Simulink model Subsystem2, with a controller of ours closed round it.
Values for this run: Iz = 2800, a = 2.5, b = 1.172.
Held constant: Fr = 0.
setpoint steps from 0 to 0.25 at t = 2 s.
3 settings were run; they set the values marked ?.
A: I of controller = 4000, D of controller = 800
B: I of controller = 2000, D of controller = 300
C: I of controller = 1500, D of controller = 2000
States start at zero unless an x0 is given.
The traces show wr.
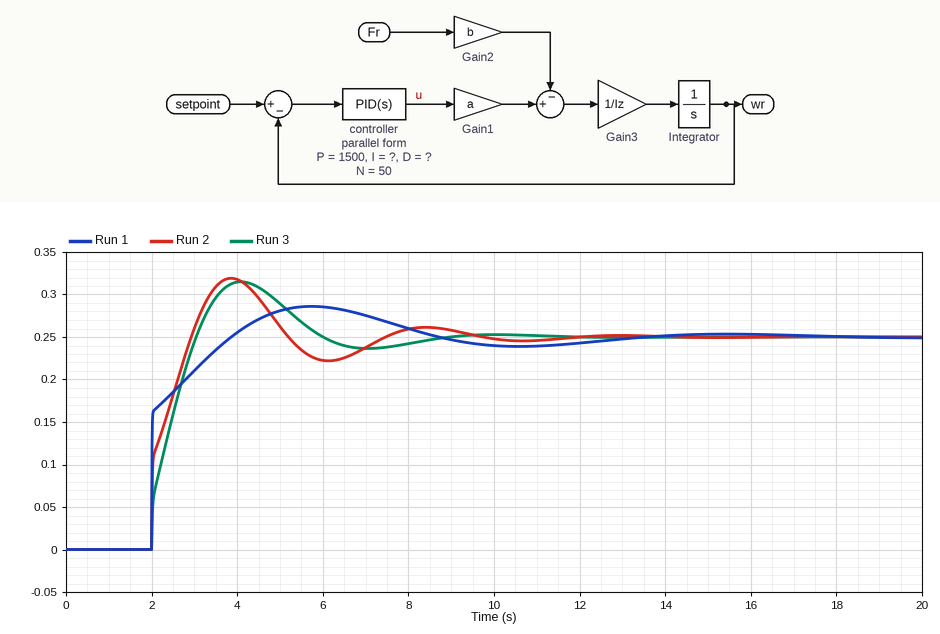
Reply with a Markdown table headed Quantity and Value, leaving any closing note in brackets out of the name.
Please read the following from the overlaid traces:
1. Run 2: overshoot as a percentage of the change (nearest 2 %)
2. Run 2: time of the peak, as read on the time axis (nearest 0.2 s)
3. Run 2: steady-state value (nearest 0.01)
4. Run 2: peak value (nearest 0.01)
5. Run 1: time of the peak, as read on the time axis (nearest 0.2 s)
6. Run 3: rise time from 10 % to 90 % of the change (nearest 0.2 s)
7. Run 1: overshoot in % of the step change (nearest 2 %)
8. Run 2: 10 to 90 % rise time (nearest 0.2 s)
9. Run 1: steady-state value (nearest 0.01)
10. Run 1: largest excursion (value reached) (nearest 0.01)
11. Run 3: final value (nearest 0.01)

| Quantity | Value |
|---|---|
| Run 2: overshoot as a percentage of the change | 28 % |
| Run 2: time of the peak, as read on the time axis | 3.8 s |
| Run 2: steady-state value | 0.25 |
| Run 2: peak value | 0.32 |
| Run 1: time of the peak, as read on the time axis | 5.8 s |
| Run 3: rise time from 10 % to 90 % of the change | 0.8 s |
| Run 1: overshoot in % of the step change | 14 % |
| Run 2: 10 to 90 % rise time | 0.8 s |
| Run 1: steady-state value | 0.25 |
| Run 1: largest excursion (value reached) | 0.29 |
| Run 3: final value | 0.25 |
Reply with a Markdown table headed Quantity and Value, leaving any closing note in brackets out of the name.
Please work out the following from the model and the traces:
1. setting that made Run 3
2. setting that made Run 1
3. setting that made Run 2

| Quantity | Value |
|---|---|
| setting that made Run 3 | B |
| setting that made Run 1 | C |
| setting that made Run 2 | A |
